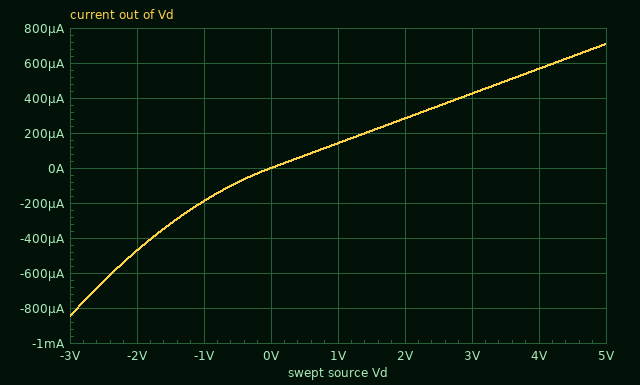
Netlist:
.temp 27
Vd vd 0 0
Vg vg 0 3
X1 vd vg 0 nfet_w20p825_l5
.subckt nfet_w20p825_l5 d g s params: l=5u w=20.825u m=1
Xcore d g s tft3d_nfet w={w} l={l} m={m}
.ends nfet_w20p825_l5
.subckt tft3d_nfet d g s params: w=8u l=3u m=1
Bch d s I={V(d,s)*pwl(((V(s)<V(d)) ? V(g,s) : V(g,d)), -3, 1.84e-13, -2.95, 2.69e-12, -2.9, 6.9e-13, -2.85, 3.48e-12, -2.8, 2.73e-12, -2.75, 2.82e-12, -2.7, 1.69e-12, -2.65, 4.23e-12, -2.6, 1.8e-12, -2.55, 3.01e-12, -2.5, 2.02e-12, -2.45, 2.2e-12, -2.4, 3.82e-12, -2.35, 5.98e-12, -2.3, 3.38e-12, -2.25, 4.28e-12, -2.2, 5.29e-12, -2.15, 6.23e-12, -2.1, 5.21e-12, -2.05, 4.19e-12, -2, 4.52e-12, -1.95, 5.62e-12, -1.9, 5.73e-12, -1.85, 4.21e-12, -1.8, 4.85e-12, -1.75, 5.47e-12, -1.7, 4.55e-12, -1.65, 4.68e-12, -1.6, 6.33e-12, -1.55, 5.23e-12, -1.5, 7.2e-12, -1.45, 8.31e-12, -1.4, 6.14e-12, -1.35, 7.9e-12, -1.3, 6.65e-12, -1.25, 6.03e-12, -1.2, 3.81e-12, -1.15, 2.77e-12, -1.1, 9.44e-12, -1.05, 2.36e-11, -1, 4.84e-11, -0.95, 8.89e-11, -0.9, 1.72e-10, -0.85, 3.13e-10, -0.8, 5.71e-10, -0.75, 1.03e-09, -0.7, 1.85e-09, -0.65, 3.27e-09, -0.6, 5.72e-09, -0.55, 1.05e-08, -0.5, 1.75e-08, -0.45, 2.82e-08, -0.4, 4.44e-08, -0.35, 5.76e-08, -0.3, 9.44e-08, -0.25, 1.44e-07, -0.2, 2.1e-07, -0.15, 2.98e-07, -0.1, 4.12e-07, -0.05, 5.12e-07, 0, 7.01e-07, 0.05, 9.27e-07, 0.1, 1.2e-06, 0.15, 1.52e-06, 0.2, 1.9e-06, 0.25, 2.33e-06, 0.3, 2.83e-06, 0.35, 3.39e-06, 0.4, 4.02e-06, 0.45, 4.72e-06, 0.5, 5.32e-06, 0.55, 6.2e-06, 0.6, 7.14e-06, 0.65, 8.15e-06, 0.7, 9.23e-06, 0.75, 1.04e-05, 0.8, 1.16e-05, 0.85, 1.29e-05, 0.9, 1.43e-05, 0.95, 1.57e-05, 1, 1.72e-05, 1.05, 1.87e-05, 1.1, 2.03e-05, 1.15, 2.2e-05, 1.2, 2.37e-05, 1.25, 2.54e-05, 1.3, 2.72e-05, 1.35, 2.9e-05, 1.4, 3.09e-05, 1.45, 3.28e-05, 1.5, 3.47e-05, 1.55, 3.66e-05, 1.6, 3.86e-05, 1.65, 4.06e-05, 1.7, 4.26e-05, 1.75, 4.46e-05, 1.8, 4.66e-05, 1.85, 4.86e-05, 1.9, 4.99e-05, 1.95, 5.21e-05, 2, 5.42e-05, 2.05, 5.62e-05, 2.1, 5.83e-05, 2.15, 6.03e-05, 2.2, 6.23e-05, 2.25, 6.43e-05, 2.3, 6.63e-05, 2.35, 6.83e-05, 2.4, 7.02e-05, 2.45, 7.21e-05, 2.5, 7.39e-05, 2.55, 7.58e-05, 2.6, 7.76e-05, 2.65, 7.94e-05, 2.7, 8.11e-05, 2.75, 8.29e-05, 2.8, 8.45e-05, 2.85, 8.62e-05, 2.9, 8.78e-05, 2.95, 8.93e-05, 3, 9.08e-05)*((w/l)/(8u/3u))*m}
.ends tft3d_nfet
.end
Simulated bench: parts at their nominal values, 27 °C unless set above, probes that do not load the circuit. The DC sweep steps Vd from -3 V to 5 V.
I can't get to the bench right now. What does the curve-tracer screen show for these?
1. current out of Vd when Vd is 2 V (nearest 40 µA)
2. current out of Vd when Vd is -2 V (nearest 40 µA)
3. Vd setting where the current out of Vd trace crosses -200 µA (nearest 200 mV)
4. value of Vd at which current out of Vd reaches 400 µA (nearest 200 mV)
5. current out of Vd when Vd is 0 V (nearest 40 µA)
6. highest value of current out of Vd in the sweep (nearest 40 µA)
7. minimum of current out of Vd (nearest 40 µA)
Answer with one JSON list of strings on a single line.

["280 µA", "-480 µA", "-1.0 V", "2.8 V", "0 A", "720 µA", "-840 µA"]
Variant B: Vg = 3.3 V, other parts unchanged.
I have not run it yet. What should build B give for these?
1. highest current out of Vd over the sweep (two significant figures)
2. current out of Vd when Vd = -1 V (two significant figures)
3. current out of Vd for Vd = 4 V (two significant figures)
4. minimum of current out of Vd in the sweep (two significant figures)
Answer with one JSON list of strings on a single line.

["780 µA", "-200 µA", "620 µA", "-890 µA"]
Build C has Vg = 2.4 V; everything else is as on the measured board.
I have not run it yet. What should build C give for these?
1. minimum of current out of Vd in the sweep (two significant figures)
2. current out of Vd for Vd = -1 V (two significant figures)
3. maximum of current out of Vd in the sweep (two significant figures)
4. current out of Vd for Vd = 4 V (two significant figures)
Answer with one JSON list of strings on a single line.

["-760 µA", "-160 µA", "550 µA", "440 µA"]
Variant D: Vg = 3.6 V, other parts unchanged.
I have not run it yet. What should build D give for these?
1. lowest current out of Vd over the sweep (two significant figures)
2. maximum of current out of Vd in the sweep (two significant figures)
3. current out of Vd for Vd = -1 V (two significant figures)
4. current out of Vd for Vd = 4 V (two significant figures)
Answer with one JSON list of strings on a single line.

["-930 µA", "850 µA", "-220 µA", "680 µA"]
